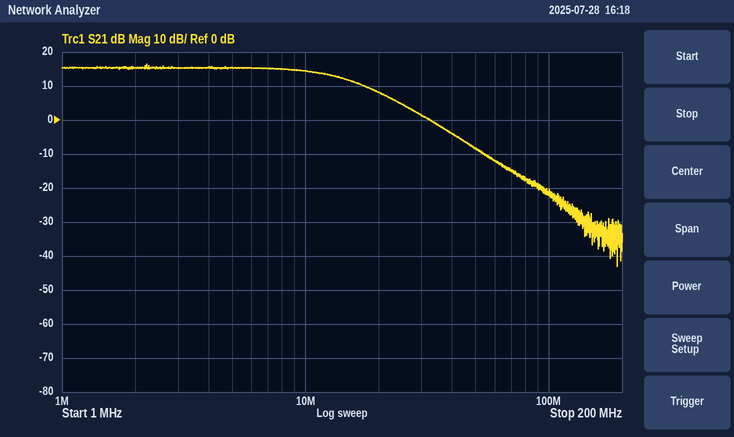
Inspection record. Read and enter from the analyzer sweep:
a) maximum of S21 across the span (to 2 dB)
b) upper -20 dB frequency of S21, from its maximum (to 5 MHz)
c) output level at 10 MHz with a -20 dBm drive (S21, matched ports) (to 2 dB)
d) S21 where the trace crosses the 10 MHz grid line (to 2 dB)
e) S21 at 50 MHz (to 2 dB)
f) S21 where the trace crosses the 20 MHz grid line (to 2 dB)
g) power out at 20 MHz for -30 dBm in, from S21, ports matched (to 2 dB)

16 dB
40 MHz
-6 dBm
14 dB
-8 dB
8 dB
-22 dBm
